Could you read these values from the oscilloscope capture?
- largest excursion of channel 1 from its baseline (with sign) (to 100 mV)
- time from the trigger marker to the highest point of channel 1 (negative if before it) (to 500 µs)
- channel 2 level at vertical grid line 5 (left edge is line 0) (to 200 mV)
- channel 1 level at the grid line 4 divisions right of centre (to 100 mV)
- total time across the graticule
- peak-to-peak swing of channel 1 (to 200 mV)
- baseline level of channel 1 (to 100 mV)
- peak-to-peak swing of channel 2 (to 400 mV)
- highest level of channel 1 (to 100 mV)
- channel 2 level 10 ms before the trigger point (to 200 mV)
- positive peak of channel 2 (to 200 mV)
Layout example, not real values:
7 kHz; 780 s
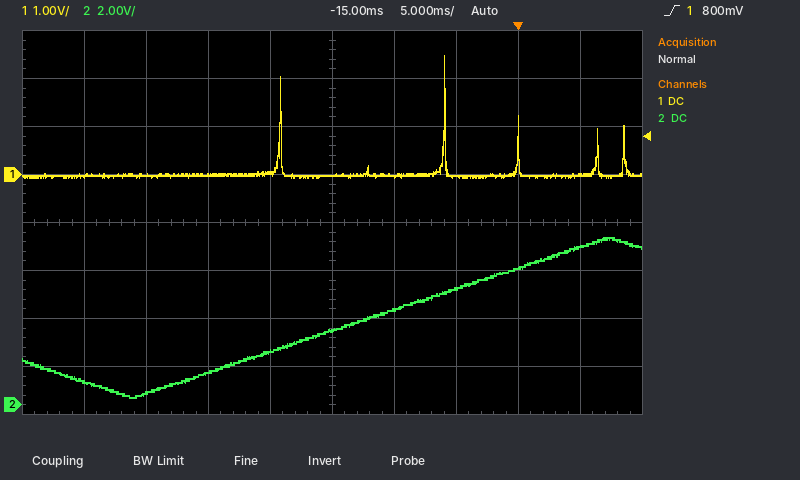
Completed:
+2.5 V; -6.0 ms; 3.2 V; 0.0 V; 50 ms; 2.6 V; 0.0 V; 6.8 V; 2.5 V; 4.0 V; 7.0 V
